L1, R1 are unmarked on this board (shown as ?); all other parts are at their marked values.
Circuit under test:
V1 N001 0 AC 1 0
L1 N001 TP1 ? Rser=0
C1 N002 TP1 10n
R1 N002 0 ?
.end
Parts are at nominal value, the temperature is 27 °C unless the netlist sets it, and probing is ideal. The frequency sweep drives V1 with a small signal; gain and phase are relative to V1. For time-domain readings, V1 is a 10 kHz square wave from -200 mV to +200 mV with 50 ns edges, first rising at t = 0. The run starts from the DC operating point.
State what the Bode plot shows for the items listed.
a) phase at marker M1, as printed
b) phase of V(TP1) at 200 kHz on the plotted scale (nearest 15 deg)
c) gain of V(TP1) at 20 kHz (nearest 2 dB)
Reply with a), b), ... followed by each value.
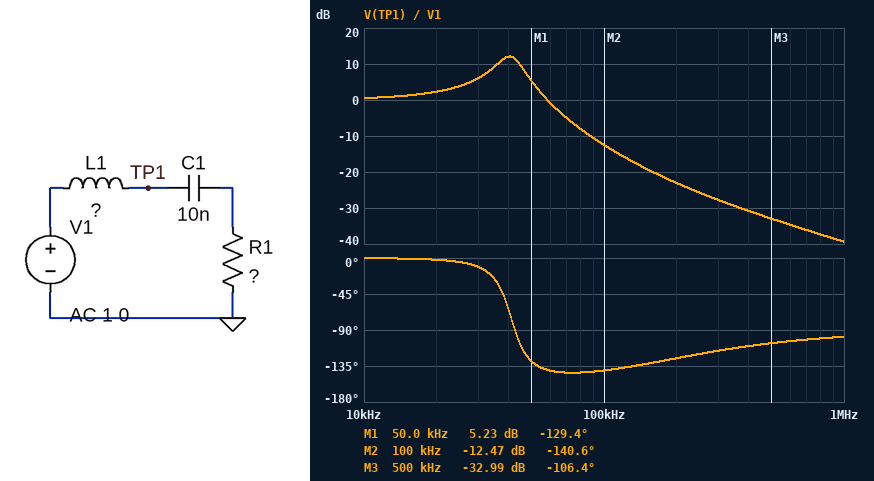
a) -129.4 deg
b) -120 deg
c) 2 dB
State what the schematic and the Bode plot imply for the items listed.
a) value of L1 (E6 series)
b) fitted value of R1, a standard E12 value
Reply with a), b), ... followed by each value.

a) 1.5 mH
b) 100 Ω
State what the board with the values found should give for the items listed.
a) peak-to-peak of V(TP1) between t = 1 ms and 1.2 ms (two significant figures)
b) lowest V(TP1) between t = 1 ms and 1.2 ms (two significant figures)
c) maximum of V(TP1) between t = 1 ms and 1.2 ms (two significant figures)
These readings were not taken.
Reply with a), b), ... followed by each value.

a) 860 mV
b) -430 mV
c) 430 mV
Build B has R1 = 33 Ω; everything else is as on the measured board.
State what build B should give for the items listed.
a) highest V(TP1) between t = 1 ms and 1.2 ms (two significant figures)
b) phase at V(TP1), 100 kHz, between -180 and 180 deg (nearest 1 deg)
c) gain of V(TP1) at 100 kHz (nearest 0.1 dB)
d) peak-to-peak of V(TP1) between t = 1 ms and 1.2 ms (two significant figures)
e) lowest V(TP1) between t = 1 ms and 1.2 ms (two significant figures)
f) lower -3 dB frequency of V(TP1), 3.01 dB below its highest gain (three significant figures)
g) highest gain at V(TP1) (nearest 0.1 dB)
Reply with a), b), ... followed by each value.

a) 420 mV
b) -166 deg
c) -13.7 dB
d) 850 mV
e) -420 mV
f) 39.2 kHz
g) 21.4 dB
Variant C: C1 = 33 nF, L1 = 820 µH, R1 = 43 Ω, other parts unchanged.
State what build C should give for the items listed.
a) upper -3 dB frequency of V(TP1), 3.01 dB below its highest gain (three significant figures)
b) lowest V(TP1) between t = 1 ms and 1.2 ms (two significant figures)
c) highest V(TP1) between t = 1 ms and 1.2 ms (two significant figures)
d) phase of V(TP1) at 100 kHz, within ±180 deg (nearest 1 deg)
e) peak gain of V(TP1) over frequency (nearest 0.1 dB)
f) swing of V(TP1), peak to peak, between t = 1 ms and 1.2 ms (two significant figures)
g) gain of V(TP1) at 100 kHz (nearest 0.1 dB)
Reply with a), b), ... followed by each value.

a) 34.0 kHz
b) -570 mV
c) 570 mV
d) -133 deg
e) 11.7 dB
f) 1.1 V
g) -17.2 dB
